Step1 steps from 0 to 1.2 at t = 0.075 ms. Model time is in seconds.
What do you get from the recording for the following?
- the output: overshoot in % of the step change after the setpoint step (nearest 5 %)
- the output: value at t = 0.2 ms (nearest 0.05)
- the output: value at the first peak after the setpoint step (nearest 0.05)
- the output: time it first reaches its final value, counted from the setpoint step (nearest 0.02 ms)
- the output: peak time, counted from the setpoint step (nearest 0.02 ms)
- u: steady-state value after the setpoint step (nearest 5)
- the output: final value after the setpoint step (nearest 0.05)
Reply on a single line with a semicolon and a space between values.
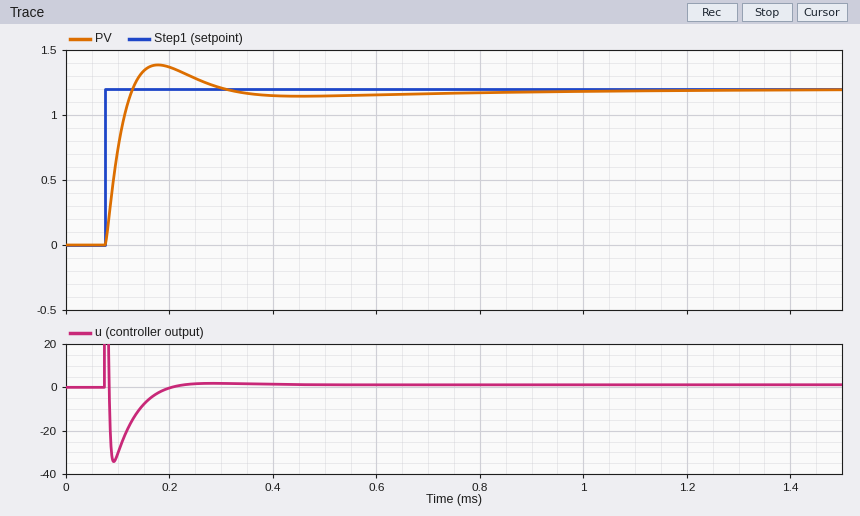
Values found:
15 %; 1.35; 1.40; 0.06 ms; 0.10 ms; 0; 1.20
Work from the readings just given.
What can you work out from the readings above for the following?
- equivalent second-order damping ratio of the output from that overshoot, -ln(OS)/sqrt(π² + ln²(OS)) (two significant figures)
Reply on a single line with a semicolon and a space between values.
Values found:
0.52
